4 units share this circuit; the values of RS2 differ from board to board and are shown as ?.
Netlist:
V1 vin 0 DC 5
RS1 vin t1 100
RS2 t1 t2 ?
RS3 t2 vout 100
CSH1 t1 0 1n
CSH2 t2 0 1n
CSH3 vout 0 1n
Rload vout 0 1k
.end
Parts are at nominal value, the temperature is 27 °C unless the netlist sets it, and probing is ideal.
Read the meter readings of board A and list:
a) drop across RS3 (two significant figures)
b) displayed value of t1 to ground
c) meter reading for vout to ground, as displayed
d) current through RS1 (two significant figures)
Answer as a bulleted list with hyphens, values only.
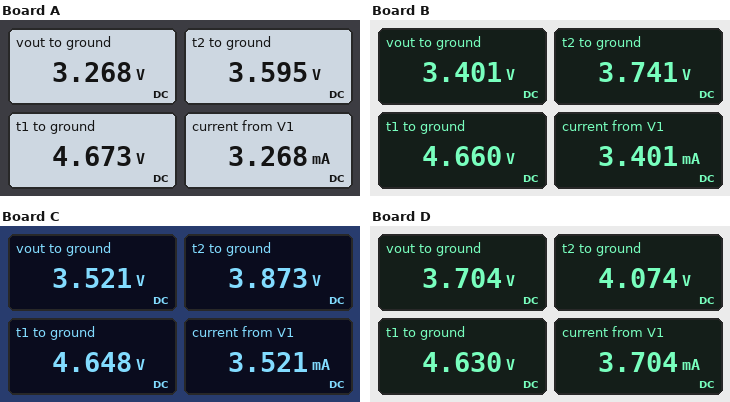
- 330 mV
- 4.673 V
- 3.268 V
- 3.3 mA
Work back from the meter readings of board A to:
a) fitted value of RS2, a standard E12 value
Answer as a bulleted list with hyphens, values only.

- 330 Ω
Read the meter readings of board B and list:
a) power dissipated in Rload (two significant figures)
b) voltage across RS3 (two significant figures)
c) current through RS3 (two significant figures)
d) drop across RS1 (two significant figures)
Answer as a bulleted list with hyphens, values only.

- 12 mW
- 340 mV
- 3.4 mA
- 340 mV
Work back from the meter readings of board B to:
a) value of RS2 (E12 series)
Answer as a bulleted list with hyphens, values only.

- 270 Ω
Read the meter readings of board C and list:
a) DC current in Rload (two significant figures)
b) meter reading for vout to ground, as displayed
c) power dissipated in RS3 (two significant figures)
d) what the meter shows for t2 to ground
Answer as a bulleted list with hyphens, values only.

- 3.5 mA
- 3.521 V
- 1.2 mW
- 3.873 V
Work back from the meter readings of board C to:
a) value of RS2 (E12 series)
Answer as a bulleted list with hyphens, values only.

- 220 Ω
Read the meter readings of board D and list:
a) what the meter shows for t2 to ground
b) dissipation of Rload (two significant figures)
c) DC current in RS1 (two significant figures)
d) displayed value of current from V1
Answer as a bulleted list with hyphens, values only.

- 4.074 V
- 14 mW
- 3.7 mA
- 3.704 mA
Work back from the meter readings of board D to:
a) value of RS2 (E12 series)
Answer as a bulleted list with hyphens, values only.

- 150 Ω
